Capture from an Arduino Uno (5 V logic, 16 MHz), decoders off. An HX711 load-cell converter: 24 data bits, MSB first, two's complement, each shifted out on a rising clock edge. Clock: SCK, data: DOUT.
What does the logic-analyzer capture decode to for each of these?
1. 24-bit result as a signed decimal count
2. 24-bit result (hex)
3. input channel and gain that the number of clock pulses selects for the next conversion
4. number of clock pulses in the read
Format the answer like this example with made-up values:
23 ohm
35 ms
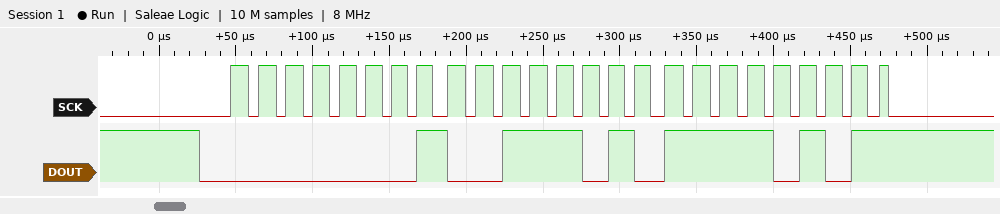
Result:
80629
0x013AF5
channel A, gain 128
25
